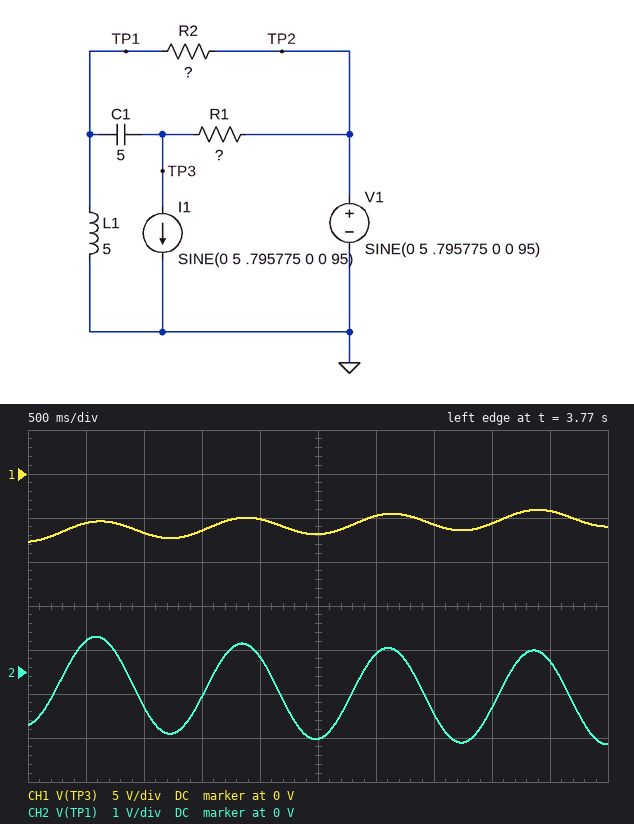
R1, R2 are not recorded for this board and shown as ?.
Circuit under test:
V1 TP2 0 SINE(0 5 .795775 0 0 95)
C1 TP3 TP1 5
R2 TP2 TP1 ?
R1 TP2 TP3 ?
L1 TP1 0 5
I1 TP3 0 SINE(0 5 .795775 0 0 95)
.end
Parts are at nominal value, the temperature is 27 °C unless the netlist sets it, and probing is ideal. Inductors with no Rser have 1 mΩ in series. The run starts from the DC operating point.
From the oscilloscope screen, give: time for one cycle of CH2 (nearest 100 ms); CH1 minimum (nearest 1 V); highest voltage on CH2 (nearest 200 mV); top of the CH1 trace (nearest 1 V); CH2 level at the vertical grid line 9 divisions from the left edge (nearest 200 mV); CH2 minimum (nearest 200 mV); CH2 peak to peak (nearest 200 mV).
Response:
1.3 s
-8 V
800 mV
-4 V
200 mV
-1.6 V
2.4 V
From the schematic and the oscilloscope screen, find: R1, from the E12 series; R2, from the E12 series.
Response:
2.7 Ω
2.2 Ω
